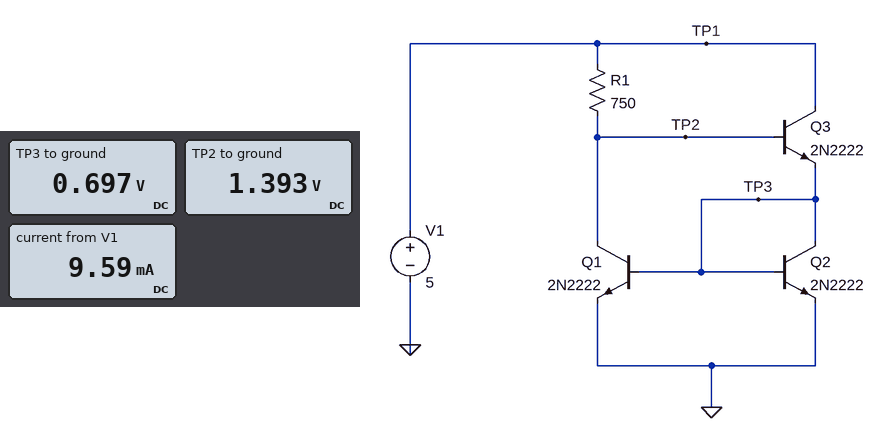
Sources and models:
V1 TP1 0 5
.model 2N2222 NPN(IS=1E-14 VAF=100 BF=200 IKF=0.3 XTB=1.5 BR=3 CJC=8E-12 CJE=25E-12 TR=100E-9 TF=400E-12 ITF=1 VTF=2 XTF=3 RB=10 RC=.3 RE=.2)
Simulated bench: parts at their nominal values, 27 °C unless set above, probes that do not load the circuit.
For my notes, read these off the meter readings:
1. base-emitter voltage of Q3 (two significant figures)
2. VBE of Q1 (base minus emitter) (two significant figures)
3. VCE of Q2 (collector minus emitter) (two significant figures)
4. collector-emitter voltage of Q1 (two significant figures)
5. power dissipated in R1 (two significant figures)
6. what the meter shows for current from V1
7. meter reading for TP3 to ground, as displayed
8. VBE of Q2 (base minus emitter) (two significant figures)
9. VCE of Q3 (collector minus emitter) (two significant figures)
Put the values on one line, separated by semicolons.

700 mV; 700 mV; 700 mV; 1.4 V; 17 mW; 9.59 mA; 0.697 V; 700 mV; 4.3 V
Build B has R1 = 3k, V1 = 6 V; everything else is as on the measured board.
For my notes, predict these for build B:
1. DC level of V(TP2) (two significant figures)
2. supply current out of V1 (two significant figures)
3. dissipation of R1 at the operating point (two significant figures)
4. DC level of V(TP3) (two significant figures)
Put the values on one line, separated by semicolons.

1.3 V; 3.1 mA; 7.3 mW; 670 mV
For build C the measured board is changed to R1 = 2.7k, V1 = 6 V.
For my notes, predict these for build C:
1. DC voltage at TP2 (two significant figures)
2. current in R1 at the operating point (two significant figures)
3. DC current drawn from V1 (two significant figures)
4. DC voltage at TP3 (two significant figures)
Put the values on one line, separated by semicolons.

1.3 V; 1.7 mA; 3.4 mA; 670 mV
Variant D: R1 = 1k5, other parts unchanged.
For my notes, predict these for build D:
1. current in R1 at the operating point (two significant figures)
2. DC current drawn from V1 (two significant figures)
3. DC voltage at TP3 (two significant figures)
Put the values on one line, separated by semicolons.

2.4 mA; 4.8 mA; 680 mV
